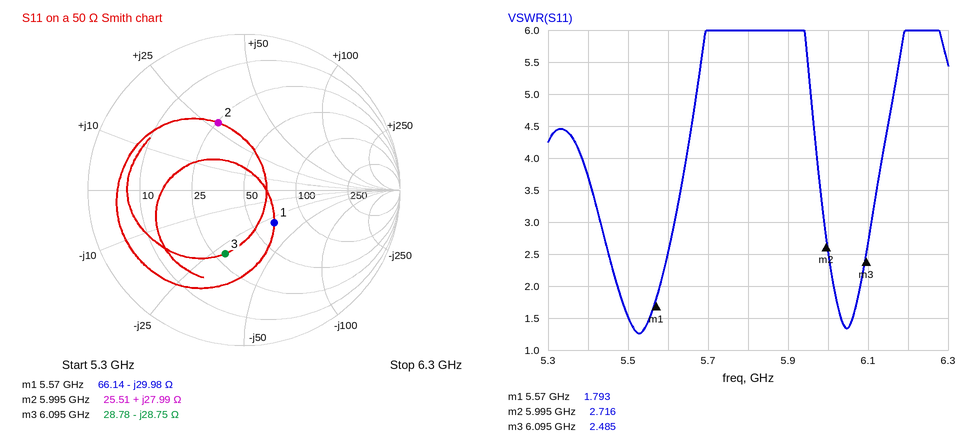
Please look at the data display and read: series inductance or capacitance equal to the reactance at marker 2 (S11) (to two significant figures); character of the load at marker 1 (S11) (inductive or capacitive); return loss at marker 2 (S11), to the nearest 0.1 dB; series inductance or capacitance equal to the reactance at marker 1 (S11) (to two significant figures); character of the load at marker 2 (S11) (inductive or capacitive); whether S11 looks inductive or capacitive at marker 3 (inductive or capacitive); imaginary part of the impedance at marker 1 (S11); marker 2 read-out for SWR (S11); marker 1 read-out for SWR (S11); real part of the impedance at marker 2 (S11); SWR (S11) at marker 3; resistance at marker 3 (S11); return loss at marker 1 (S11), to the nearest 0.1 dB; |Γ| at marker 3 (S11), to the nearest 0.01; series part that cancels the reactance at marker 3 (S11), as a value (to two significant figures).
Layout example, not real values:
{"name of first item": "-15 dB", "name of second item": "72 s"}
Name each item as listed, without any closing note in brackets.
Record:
{"series inductance or capacitance equal to the reactance at marker 2 (S11)": "740 pH", "character of the load at marker 1 (S11)": "capacitive", "return loss at marker 2 (S11), to the nearest 0.1 dB": "6.7 dB", "series inductance or capacitance equal to the reactance at marker 1 (S11)": "950 fF", "character of the load at marker 2 (S11)": "inductive", "whether S11 looks inductive or capacitive at marker 3": "capacitive", "imaginary part of the impedance at marker 1": "-29.98 Ω", "marker 2 read-out for SWR": "2.716", "marker 1 read-out for SWR": "1.793", "real part of the impedance at marker 2": "25.51 Ω", "SWR (S11) at marker 3": "2.485", "resistance at marker 3": "28.78 Ω", "return loss at marker 1 (S11), to the nearest 0.1 dB": "10.9 dB", "|Γ| at marker 3 (S11), to the nearest 0.01": "0.43", "series part that cancels the reactance at marker 3 (S11), as a value": "750 pH"}
